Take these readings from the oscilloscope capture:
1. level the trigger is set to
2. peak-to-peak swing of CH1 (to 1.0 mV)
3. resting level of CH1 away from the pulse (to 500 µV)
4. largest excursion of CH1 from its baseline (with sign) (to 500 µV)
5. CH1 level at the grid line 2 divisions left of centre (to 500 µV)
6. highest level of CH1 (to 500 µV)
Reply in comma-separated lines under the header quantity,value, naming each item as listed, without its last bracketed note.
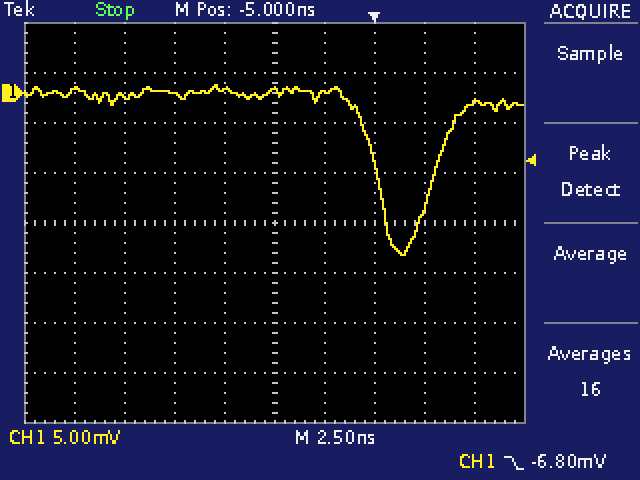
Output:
quantity,value
level the trigger is set to,-6.80 mV
peak-to-peak swing of CH1,17.0 mV
resting level of CH1 away from the pulse,0.0 mV
largest excursion of CH1 from its baseline (with sign),-16.0 mV
CH1 level at the grid line 2 divisions left of centre,0.0 mV
highest level of CH1,1.0 mV
